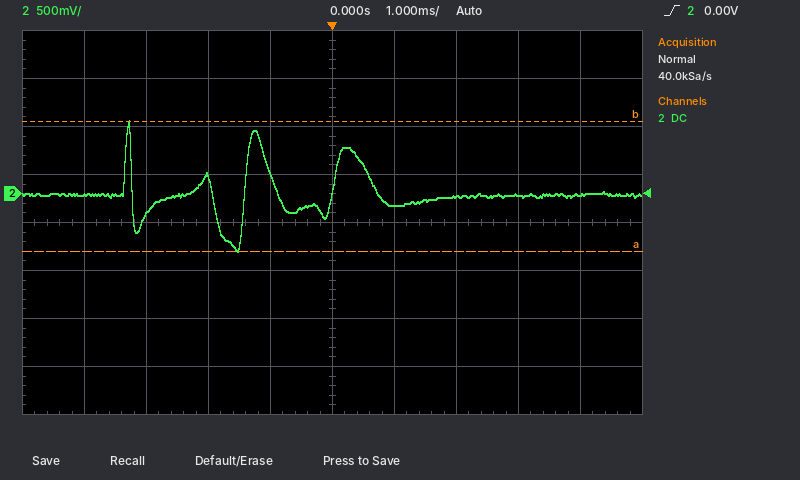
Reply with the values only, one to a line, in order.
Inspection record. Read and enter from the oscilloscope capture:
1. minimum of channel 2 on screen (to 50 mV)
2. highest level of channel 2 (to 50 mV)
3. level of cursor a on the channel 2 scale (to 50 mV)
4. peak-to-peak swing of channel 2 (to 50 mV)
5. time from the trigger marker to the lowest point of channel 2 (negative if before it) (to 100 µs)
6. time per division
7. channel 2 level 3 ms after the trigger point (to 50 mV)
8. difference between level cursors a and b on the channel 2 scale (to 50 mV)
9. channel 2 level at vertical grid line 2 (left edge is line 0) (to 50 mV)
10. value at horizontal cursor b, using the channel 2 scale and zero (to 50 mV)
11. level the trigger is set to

-600 mV
750 mV
-600 mV
1.35 V
-1.5 ms
1 ms
0 mV
1.35 V
-200 mV
750 mV
0.00 V
